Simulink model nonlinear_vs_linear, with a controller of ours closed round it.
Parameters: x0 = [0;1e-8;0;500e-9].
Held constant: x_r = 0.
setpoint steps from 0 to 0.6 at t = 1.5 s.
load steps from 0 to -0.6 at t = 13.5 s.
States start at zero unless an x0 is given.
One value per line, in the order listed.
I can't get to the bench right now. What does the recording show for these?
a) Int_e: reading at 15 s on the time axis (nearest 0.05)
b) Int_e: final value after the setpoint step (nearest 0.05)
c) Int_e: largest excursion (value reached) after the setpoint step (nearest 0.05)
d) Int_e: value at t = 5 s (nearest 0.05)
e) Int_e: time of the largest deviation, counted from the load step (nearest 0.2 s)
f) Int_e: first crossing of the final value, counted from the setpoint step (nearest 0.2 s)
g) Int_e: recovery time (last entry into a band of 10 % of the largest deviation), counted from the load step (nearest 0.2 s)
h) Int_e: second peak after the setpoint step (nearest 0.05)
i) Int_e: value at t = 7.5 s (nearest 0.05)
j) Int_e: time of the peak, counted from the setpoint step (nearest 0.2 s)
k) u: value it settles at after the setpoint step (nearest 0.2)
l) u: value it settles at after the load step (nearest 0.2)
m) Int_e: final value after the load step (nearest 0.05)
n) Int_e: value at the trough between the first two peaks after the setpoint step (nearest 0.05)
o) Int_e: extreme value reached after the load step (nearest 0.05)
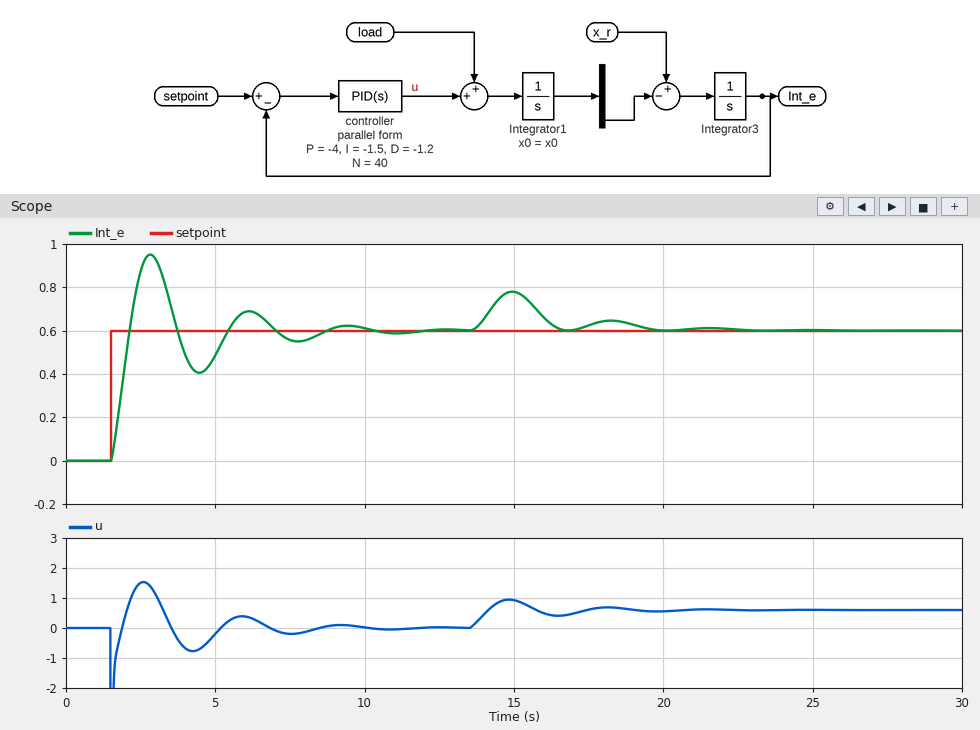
0.80
0.60
0.95
0.50
1.4 s
0.6 s
5.8 s
0.70
0.55
1.4 s
0.0
0.6
0.60
0.40
0.80
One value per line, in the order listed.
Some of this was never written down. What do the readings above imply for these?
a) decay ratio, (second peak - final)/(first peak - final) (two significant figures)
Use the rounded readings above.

0.29
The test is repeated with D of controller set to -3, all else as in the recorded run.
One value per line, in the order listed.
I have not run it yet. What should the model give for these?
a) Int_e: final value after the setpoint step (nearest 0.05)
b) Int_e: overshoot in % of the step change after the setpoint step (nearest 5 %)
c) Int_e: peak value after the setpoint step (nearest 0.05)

0.60
25 %
0.75
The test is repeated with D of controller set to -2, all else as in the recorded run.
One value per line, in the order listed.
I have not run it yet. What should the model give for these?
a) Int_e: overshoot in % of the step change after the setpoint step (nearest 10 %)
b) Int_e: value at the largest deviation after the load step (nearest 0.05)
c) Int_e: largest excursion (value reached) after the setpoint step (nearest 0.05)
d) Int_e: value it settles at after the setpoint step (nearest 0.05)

40 %
0.75
0.85
0.60
